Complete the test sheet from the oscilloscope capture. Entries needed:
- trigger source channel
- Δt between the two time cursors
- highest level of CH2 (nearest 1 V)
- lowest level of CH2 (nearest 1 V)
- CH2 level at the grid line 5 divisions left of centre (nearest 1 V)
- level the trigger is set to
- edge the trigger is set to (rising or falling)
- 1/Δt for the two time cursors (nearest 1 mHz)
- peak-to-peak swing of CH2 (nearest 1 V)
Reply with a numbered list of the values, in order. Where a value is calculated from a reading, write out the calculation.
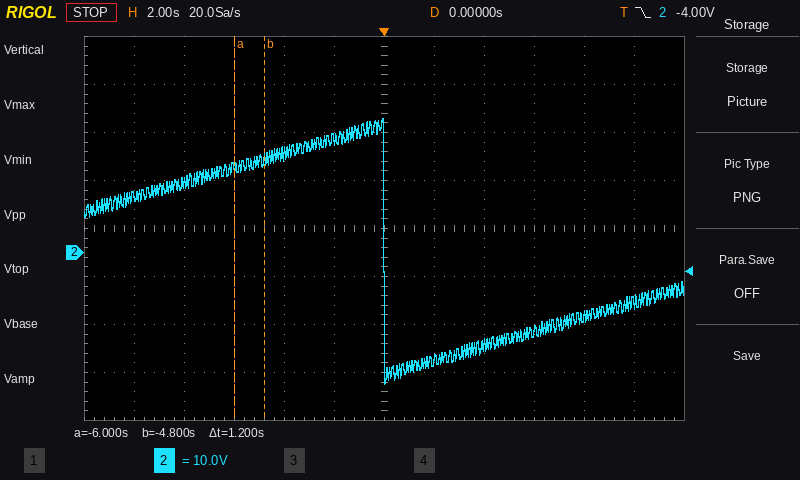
1. CH2
2. 1.2 s
3. 28 V
4. -27 V
5. 12 V
6. -4.00 V
7. falling
8. 1 / 1.2 s ≈ 833 mHz
9. 28 V − (-27 V) = 55 V
